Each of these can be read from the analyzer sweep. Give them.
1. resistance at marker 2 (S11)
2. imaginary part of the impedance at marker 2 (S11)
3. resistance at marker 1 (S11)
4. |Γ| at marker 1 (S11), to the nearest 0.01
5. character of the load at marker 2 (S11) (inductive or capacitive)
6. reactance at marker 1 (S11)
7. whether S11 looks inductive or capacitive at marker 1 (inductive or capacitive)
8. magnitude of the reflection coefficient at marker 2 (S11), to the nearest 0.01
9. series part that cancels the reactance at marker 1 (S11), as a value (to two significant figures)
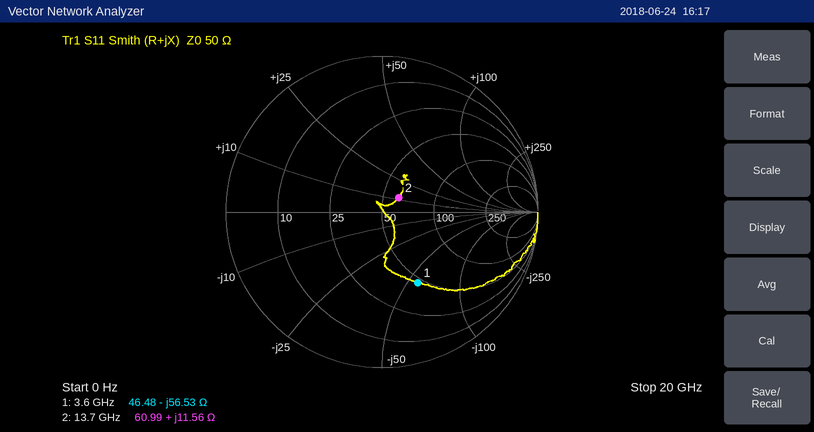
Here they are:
60.99 Ω
+11.56 Ω
46.48 Ω
0.51
inductive
-56.53 Ω
capacitive
0.14
2.5 nH
